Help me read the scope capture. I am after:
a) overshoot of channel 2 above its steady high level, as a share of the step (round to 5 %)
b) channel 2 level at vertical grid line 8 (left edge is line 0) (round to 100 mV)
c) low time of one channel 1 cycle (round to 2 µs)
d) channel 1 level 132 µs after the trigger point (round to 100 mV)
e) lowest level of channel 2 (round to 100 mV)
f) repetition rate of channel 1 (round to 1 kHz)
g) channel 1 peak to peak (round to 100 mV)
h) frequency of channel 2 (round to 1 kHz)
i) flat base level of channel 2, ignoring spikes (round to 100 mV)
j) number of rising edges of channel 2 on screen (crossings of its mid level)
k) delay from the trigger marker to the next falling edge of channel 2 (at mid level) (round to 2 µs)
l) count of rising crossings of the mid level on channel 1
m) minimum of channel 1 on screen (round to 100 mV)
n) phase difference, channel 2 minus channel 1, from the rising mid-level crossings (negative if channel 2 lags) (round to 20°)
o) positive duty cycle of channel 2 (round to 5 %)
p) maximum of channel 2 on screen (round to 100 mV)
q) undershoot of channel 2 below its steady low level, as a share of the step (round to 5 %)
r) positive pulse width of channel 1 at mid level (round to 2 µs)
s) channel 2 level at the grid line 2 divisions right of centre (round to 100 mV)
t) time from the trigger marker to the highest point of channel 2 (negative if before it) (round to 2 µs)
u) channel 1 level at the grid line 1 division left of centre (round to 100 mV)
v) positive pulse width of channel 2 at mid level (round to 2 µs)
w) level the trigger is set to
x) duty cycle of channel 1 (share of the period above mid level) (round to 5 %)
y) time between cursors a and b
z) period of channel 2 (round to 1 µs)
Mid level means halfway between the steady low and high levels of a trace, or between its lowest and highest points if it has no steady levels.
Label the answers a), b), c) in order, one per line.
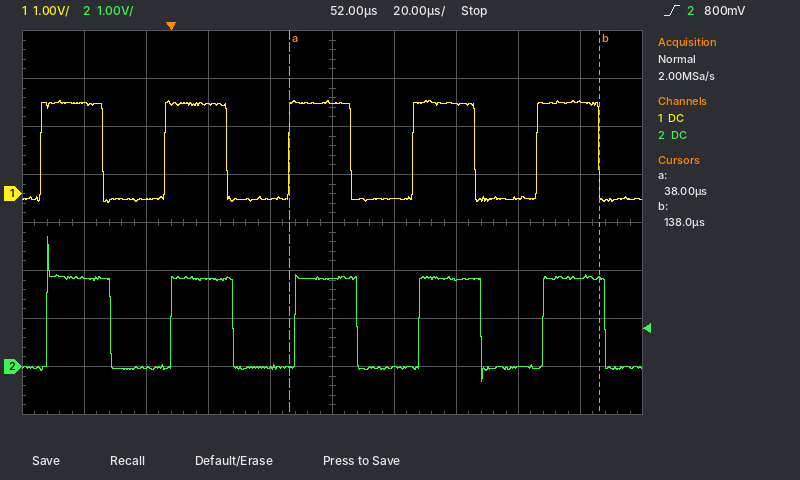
a) 45 %
b) 0.0 V
c) 20 µs
d) 1.9 V
e) -300 mV
f) 25 kHz
g) 2.1 V
h) 25 kHz
i) 0.0 V
j) 5
k) 20 µs
l) 5
m) -200 mV
n) -20°
o) 50 %
p) 2.7 V
q) 15 %
r) 20 µs
s) 1.8 V
t) -40 µs
u) -100 mV
v) 20 µs
w) 800 mV
x) 50 %
y) 100 µs
z) 40 µs
